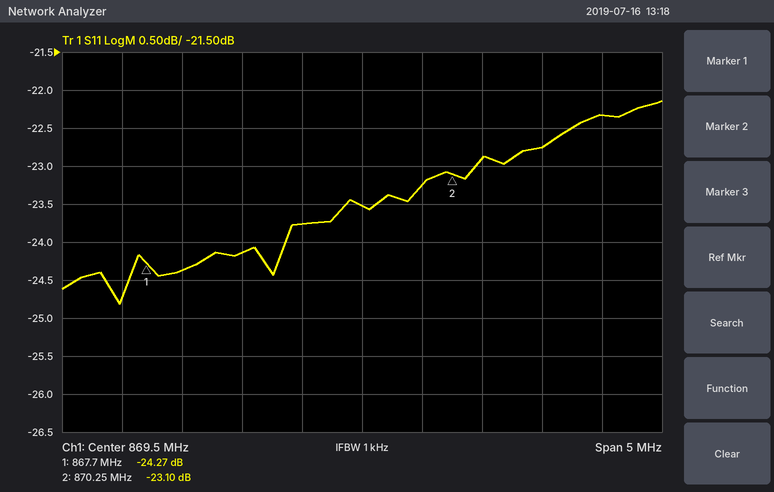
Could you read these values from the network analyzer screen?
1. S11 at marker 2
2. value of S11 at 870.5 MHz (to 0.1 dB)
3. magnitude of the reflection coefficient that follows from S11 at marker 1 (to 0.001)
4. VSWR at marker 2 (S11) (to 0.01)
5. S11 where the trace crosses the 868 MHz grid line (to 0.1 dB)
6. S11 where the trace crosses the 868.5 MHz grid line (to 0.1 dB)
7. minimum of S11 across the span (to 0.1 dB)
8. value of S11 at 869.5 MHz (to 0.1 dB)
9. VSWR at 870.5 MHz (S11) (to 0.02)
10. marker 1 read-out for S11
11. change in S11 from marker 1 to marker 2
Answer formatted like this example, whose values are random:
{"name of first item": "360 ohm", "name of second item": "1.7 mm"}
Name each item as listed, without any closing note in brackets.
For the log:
{"S11 at marker 2": "-23.10 dB", "value of S11 at 870.5 MHz": "-22.9 dB", "magnitude of the reflection coefficient that follows from S11 at marker 1": "0.061", "VSWR at marker 2 (S11)": "1.15", "S11 where the trace crosses the 868 MHz grid line": "-24.4 dB", "S11 where the trace crosses the 868.5 MHz grid line": "-24.1 dB", "minimum of S11 across the span": "-24.8 dB", "value of S11 at 869.5 MHz": "-23.5 dB", "VSWR at 870.5 MHz (S11)": "1.16", "marker 1 read-out for S11": "-24.27 dB", "change in S11 from marker 1 to marker 2": "1.17 dB"}
